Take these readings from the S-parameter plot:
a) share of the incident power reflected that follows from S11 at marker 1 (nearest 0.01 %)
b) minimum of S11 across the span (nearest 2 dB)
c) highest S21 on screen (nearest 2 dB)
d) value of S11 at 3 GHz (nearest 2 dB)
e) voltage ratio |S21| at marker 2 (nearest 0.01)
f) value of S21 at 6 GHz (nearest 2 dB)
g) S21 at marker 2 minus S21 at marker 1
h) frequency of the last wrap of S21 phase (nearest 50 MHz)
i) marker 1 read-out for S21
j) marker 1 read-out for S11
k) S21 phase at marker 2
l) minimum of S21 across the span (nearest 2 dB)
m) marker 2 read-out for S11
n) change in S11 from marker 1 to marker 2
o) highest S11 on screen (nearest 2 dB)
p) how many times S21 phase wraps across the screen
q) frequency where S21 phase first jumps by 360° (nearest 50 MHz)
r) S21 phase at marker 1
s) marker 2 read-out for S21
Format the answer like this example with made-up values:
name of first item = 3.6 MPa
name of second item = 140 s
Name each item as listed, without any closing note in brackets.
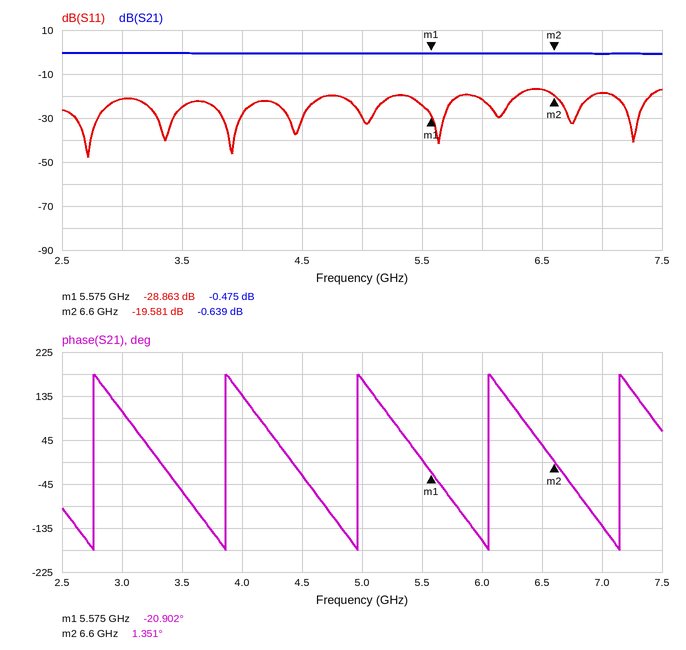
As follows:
share of the incident power reflected that follows from S11 at marker 1 = 0.13 %
minimum of S11 across the span = -48 dB
highest S21 on screen = 0 dB
value of S11 at 3 GHz = -22 dB
voltage ratio |S21| at marker 2 = 0.93
value of S21 at 6 GHz = 0 dB
S21 at marker 2 minus S21 at marker 1 = -0.164 dB
frequency of the last wrap of S21 phase = 7.15 GHz
marker 1 read-out for S21 = -0.475 dB
marker 1 read-out for S11 = -28.863 dB
S21 phase at marker 2 = 1.351°
minimum of S21 across the span = 0 dB
marker 2 read-out for S11 = -19.581 dB
change in S11 from marker 1 to marker 2 = 9.282 dB
highest S11 on screen = -16 dB
how many times S21 phase wraps across the screen = 5
frequency where S21 phase first jumps by 360° = 2.75 GHz
S21 phase at marker 1 = -20.902°
marker 2 read-out for S21 = -0.639 dB
